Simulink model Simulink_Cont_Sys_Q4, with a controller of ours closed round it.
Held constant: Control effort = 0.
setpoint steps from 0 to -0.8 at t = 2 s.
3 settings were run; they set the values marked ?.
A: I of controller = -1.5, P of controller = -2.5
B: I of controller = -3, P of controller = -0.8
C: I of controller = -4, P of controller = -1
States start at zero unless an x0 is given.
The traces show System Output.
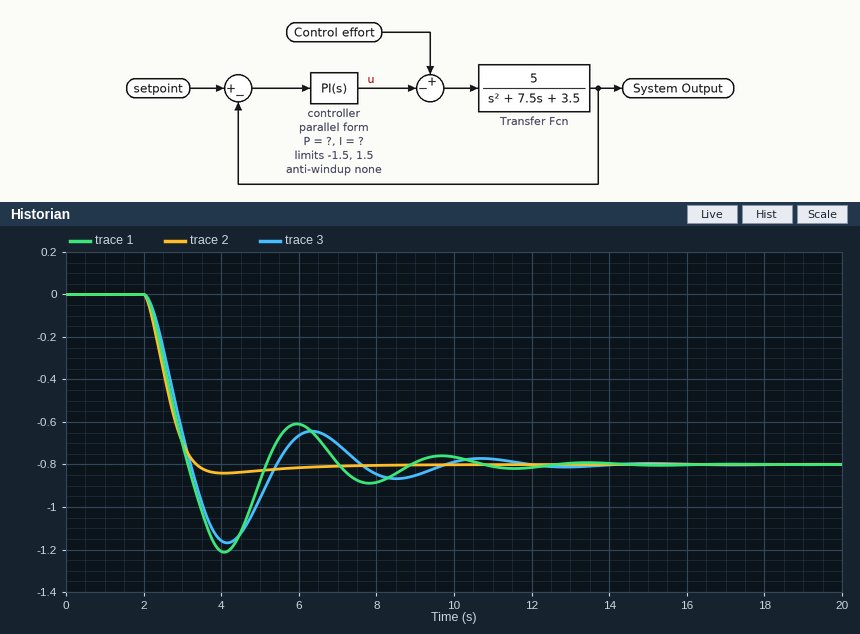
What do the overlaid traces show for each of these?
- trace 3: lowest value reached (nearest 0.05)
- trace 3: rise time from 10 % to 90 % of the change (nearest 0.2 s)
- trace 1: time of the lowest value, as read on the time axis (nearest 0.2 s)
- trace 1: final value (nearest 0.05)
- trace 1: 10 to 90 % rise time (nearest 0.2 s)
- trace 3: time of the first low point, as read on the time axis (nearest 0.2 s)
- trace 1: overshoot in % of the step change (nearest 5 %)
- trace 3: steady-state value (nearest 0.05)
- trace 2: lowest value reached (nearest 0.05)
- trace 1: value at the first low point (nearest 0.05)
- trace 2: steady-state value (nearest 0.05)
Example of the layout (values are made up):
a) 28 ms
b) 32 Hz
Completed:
a) -1.15
b) 0.8 s
c) 4.0 s
d) -0.80
e) 0.8 s
f) 4.2 s
g) 50 %
h) -0.80
i) -0.85
j) -1.20
k) -0.80
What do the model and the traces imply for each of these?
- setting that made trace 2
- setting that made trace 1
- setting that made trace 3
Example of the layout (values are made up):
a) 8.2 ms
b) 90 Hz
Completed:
a) A
b) C
c) B
